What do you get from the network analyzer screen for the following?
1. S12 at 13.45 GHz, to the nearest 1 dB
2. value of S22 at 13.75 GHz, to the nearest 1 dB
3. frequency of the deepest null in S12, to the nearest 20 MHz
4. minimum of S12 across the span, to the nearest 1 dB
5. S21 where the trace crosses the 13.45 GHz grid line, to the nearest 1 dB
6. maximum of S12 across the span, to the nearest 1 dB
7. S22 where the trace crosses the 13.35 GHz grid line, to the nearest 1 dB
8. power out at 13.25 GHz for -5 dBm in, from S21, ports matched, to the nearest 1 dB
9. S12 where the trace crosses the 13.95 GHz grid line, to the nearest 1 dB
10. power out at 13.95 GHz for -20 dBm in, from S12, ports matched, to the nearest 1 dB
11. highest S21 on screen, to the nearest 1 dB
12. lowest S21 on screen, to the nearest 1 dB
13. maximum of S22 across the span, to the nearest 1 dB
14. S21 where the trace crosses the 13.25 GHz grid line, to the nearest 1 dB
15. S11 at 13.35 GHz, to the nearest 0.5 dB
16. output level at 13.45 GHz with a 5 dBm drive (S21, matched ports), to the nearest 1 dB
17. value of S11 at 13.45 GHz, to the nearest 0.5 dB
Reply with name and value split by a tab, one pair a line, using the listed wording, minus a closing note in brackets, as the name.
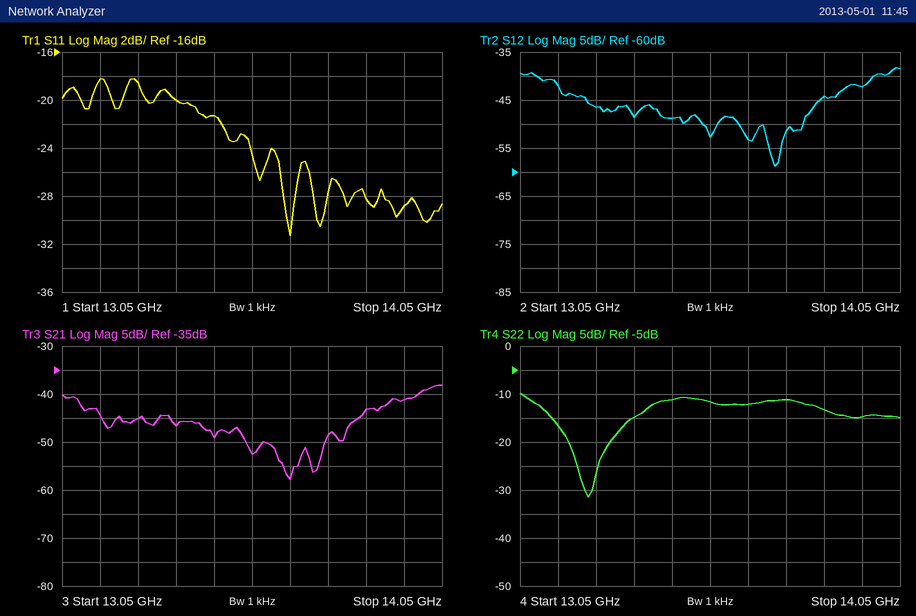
S12 at 13.45 GHz, to the nearest 1 dB	-49 dB
value of S22 at 13.75 GHz, to the nearest 1 dB	-11 dB
frequency of the deepest null in S12, to the nearest 20 MHz	13.72 GHz
minimum of S12 across the span, to the nearest 1 dB	-59 dB
S21 where the trace crosses the 13.45 GHz grid line, to the nearest 1 dB	-49 dB
maximum of S12 across the span, to the nearest 1 dB	-38 dB
S22 where the trace crosses the 13.35 GHz grid line, to the nearest 1 dB	-15 dB
power out at 13.25 GHz for -5 dBm in, from S21, ports matched, to the nearest 1 dB	-50 dBm
S12 where the trace crosses the 13.95 GHz grid line, to the nearest 1 dB	-42 dB
power out at 13.95 GHz for -20 dBm in, from S12, ports matched, to the nearest 1 dB	-62 dBm
highest S21 on screen, to the nearest 1 dB	-38 dB
lowest S21 on screen, to the nearest 1 dB	-58 dB
maximum of S22 across the span, to the nearest 1 dB	-10 dB
S21 where the trace crosses the 13.25 GHz grid line, to the nearest 1 dB	-45 dB
S11 at 13.35 GHz, to the nearest 0.5 dB	-20.0 dB
output level at 13.45 GHz with a 5 dBm drive (S21, matched ports), to the nearest 1 dB	-44 dBm
value of S11 at 13.45 GHz, to the nearest 0.5 dB	-21.5 dB
